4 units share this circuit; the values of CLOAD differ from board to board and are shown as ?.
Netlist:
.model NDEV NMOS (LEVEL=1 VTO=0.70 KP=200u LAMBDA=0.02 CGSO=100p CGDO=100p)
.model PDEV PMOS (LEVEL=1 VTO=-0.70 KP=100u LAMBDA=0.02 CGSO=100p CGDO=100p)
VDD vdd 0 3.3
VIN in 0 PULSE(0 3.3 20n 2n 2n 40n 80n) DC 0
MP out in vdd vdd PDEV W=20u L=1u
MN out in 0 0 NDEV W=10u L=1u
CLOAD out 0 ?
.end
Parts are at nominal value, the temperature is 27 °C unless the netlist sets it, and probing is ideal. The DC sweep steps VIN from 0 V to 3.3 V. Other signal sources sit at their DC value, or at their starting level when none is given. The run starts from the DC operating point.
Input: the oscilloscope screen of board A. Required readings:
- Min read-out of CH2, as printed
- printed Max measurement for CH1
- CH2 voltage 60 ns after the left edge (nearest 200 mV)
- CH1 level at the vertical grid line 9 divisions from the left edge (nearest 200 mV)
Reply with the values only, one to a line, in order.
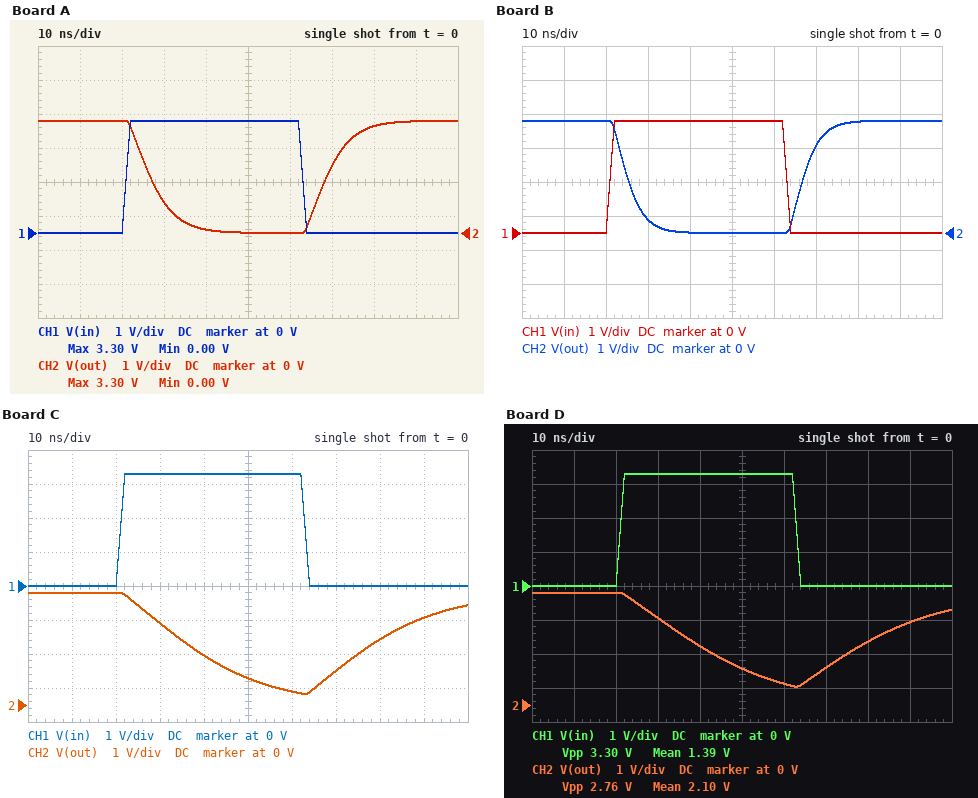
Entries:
0.00 V
3.30 V
0 V
0 V
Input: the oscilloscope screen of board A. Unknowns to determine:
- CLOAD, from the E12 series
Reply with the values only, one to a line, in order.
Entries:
22 pF
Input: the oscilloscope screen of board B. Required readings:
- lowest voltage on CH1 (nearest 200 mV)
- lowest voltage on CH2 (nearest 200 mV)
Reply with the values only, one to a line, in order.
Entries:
0 V
0 V
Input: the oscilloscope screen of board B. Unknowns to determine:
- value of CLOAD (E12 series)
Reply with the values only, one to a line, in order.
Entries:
15 pF
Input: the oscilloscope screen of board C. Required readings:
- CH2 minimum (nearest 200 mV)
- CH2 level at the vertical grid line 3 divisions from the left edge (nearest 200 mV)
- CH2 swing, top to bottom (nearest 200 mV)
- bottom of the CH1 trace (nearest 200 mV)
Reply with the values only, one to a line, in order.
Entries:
400 mV
2.4 V
3.0 V
0 V
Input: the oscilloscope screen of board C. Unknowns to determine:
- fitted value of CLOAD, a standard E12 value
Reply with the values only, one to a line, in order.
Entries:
68 pF
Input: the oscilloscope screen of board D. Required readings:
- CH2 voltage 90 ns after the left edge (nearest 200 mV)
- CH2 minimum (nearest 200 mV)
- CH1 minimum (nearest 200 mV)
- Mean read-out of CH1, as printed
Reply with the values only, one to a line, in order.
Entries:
2.4 V
600 mV
0 V
1.39 V
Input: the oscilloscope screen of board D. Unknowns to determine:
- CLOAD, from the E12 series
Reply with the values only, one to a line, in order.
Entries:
82 pF
